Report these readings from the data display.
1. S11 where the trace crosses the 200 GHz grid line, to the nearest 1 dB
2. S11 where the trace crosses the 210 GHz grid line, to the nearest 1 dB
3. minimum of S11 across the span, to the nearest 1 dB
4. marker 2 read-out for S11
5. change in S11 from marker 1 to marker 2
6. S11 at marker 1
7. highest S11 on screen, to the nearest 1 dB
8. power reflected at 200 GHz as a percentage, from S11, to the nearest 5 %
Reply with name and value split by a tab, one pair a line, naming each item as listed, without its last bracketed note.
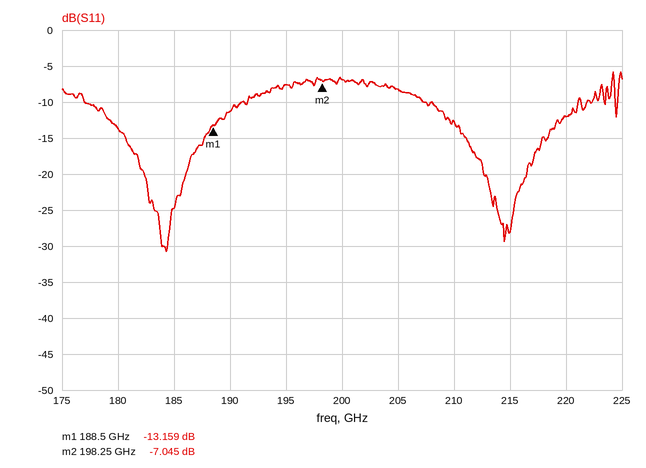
S11 where the trace crosses the 200 GHz grid line, to the nearest 1 dB	-7 dB
S11 where the trace crosses the 210 GHz grid line, to the nearest 1 dB	-13 dB
minimum of S11 across the span, to the nearest 1 dB	-31 dB
marker 2 read-out for S11	-7.045 dB
change in S11 from marker 1 to marker 2	6.114 dB
S11 at marker 1	-13.159 dB
highest S11 on screen, to the nearest 1 dB	-6 dB
power reflected at 200 GHz as a percentage, from S11, to the nearest 5 %	20 %
